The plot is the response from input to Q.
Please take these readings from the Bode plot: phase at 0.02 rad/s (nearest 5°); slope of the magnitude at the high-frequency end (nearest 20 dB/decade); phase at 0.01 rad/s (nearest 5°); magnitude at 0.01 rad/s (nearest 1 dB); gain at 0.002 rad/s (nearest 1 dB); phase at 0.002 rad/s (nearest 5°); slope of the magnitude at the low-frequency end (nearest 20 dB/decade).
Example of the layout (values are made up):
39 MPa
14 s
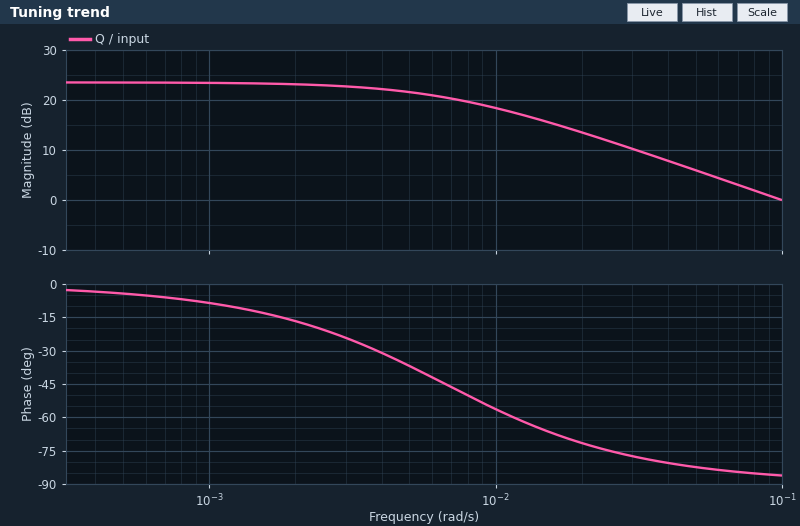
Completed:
-70°
-20 dB/decade
-55°
18 dB
23 dB
-15°
0 dB/decade
